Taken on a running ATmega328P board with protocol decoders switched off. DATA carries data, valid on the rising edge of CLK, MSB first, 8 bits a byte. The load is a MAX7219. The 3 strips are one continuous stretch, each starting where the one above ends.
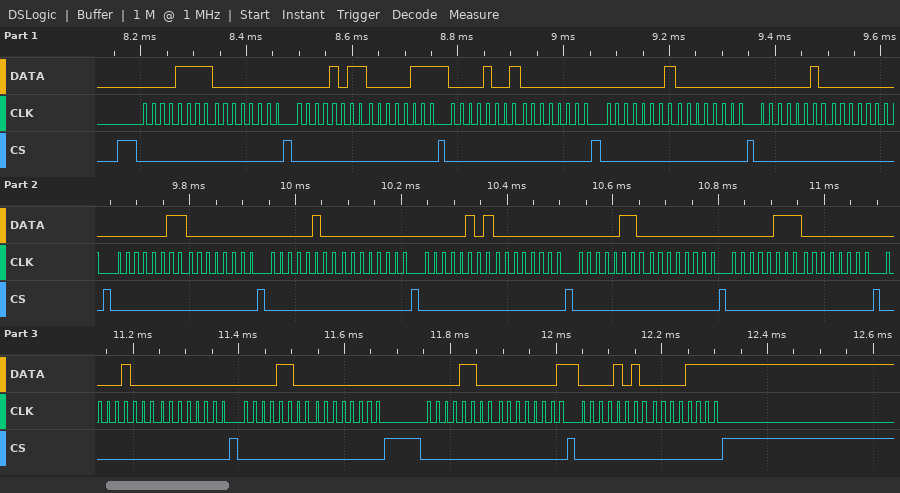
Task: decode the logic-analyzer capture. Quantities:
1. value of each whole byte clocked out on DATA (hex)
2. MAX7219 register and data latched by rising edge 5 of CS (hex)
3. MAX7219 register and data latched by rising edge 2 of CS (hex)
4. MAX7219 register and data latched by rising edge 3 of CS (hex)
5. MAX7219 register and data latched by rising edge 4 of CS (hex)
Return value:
0F 00 0B 07 09 00 01 00 02 00 03 00 04 00 05 00 06 00 07 00 08 00 0C 00 0C 01 0A 0F
register 0x1, data 0x00
register 0xF, data 0x00
register 0xB, data 0x07
register 0x9, data 0x00
